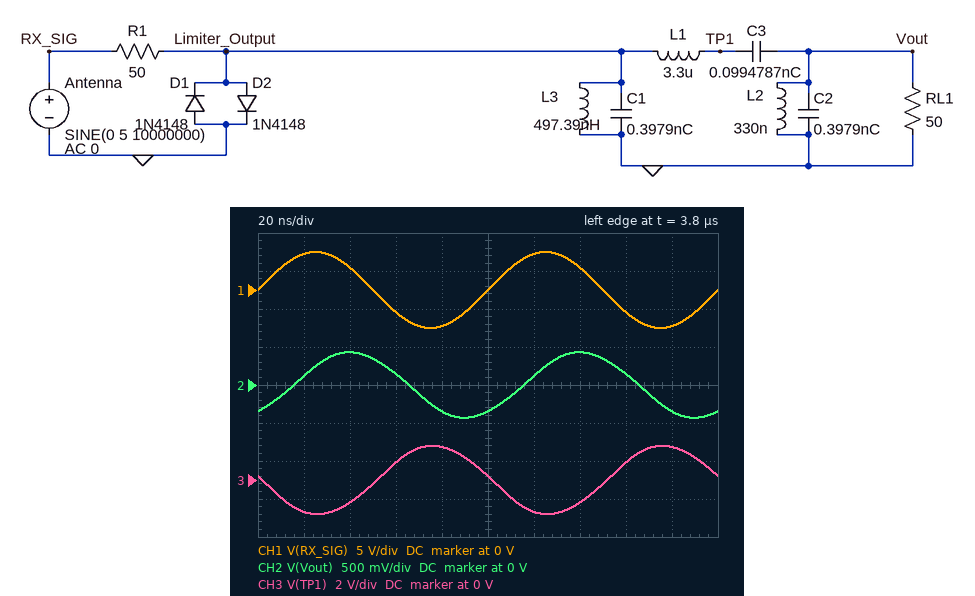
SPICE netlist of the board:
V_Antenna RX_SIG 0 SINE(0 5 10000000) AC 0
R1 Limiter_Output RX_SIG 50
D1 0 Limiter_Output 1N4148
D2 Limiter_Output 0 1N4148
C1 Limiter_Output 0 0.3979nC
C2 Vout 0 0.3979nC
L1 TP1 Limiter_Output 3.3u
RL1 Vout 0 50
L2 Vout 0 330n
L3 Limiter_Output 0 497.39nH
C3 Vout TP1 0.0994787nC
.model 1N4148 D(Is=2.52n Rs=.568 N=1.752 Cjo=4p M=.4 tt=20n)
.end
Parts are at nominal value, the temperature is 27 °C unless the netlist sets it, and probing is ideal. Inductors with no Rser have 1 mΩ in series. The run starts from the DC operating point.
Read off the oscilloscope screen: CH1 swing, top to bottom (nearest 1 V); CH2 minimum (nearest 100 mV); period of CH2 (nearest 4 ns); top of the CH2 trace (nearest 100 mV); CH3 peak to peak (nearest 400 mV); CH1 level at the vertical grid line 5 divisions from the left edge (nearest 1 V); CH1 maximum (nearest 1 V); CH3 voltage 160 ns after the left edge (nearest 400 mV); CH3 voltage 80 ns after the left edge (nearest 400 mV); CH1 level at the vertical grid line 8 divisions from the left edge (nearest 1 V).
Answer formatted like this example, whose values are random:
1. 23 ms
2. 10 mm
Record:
1. 10 V
2. -400 mV
3. 100 ns
4. 400 mV
5. 3.6 V
6. 0 V
7. 5 V
8. 800 mV
9. 1.6 V
10. -3 V
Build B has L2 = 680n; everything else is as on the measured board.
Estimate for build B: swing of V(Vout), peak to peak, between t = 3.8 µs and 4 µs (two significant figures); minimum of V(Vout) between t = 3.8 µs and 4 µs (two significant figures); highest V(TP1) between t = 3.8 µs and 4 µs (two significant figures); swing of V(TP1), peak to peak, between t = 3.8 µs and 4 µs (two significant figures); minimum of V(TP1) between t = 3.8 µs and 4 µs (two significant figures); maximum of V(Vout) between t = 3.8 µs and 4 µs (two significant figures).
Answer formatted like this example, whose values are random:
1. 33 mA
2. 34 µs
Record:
1. 1.5 V
2. -740 mV
3. 2.6 V
4. 5.2 V
5. -2.6 V
6. 740 mV
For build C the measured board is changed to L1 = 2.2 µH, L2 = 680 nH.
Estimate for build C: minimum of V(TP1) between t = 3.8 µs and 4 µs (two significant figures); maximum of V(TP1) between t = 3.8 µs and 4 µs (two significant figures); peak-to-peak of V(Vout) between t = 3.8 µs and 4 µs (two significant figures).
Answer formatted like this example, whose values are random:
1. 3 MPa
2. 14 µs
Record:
1. -2.9 V
2. 2.9 V
3. 1.7 V
